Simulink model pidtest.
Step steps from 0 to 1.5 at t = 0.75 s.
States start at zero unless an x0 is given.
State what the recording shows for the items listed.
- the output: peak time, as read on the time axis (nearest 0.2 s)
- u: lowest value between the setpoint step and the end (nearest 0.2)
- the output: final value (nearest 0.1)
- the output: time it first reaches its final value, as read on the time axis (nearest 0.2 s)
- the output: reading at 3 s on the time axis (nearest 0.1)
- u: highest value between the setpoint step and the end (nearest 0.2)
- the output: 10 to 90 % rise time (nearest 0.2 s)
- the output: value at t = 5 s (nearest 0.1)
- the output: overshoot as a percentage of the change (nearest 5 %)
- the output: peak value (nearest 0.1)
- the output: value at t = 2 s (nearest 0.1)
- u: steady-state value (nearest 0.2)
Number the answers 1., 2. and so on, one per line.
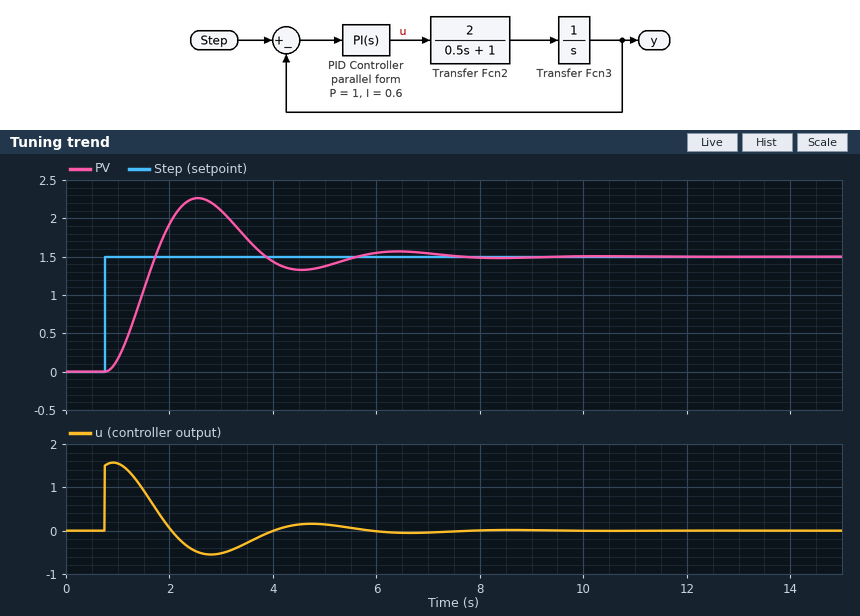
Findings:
1. 2.6 s
2. -0.6
3. 1.5
4. 1.8 s
5. 2.1
6. 1.6
7. 0.6 s
8. 1.4
9. 50 %
10. 2.3
11. 1.9
12. 0.0
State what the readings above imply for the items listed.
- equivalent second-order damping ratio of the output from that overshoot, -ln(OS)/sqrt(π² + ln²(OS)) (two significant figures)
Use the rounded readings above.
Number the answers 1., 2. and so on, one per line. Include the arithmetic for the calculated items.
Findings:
1. ln(0.5) = -0.693; 0.693 / sqrt(9.870 + 0.480) = 0.22
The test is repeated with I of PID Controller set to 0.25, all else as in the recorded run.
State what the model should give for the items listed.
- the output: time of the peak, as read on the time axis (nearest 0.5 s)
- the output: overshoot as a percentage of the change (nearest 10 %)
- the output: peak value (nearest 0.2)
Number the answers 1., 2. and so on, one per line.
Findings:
1. 2.5 s
2. 30 %
3. 2.0
